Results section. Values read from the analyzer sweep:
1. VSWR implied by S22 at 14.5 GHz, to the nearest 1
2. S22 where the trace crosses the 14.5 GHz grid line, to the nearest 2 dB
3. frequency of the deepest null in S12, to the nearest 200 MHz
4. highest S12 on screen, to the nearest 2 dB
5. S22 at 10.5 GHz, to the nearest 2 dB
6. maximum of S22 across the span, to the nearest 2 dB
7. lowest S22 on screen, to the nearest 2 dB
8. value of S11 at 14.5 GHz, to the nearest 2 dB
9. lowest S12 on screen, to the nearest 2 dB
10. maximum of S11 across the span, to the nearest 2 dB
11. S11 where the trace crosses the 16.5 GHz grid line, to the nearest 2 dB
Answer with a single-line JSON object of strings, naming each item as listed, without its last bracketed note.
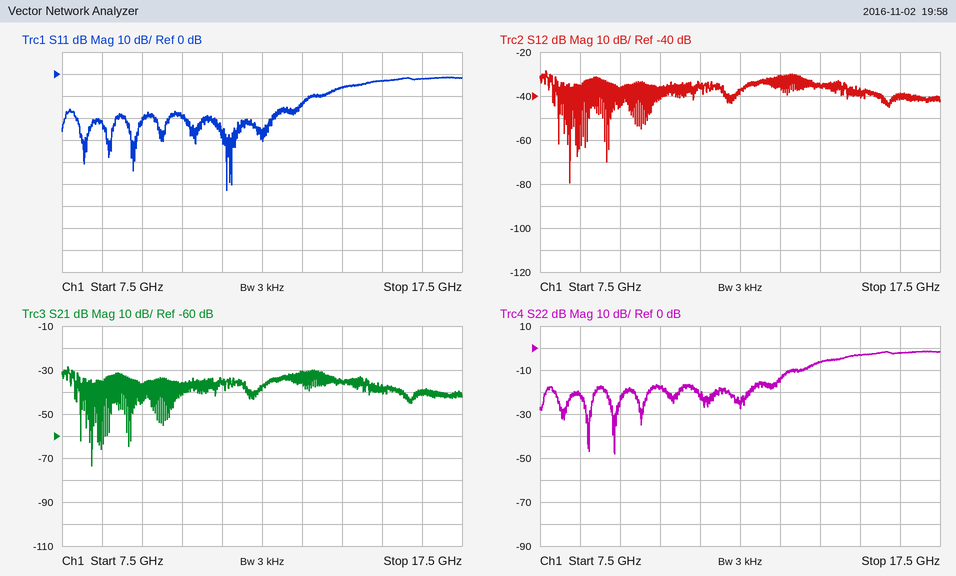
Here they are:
{"VSWR implied by S22 at 14.5 GHz, to the nearest 1": "3", "S22 where the trace crosses the 14.5 GHz grid line, to the nearest 2 dB": "-6 dB", "frequency of the deepest null in S12, to the nearest 200 MHz": "8.2 GHz", "highest S12 on screen, to the nearest 2 dB": "-28 dB", "S22 at 10.5 GHz, to the nearest 2 dB": "-18 dB", "maximum of S22 across the span, to the nearest 2 dB": "-2 dB", "lowest S22 on screen, to the nearest 2 dB": "-48 dB", "value of S11 at 14.5 GHz, to the nearest 2 dB": "-6 dB", "lowest S12 on screen, to the nearest 2 dB": "-80 dB", "maximum of S11 across the span, to the nearest 2 dB": "-2 dB", "S11 where the trace crosses the 16.5 GHz grid line, to the nearest 2 dB": "-2 dB"}
